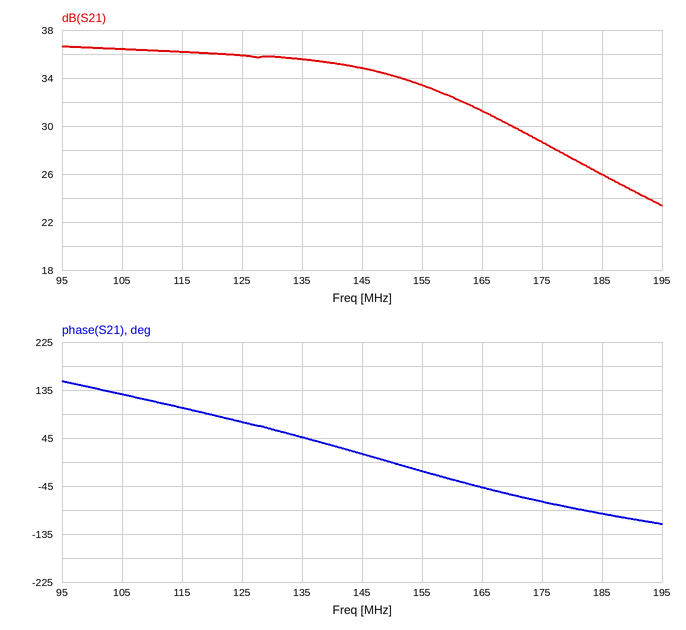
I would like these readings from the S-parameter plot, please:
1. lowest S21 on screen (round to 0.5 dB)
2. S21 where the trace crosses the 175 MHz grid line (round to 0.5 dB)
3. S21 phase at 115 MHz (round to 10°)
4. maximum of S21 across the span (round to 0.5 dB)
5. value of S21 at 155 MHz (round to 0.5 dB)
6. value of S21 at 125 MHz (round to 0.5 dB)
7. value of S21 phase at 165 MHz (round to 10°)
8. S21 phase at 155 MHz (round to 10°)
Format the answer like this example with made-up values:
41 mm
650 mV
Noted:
23.5 dB
28.5 dB
100°
36.5 dB
33.5 dB
36.0 dB
-50°
-20°
